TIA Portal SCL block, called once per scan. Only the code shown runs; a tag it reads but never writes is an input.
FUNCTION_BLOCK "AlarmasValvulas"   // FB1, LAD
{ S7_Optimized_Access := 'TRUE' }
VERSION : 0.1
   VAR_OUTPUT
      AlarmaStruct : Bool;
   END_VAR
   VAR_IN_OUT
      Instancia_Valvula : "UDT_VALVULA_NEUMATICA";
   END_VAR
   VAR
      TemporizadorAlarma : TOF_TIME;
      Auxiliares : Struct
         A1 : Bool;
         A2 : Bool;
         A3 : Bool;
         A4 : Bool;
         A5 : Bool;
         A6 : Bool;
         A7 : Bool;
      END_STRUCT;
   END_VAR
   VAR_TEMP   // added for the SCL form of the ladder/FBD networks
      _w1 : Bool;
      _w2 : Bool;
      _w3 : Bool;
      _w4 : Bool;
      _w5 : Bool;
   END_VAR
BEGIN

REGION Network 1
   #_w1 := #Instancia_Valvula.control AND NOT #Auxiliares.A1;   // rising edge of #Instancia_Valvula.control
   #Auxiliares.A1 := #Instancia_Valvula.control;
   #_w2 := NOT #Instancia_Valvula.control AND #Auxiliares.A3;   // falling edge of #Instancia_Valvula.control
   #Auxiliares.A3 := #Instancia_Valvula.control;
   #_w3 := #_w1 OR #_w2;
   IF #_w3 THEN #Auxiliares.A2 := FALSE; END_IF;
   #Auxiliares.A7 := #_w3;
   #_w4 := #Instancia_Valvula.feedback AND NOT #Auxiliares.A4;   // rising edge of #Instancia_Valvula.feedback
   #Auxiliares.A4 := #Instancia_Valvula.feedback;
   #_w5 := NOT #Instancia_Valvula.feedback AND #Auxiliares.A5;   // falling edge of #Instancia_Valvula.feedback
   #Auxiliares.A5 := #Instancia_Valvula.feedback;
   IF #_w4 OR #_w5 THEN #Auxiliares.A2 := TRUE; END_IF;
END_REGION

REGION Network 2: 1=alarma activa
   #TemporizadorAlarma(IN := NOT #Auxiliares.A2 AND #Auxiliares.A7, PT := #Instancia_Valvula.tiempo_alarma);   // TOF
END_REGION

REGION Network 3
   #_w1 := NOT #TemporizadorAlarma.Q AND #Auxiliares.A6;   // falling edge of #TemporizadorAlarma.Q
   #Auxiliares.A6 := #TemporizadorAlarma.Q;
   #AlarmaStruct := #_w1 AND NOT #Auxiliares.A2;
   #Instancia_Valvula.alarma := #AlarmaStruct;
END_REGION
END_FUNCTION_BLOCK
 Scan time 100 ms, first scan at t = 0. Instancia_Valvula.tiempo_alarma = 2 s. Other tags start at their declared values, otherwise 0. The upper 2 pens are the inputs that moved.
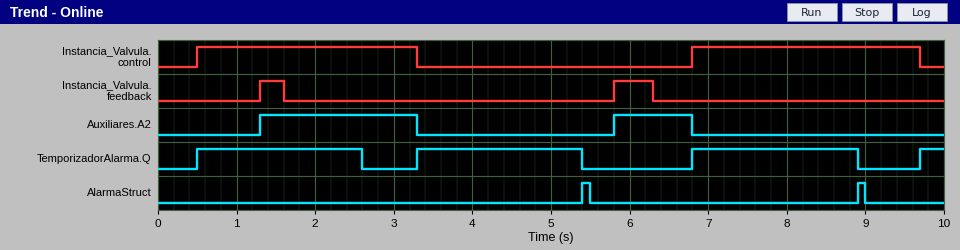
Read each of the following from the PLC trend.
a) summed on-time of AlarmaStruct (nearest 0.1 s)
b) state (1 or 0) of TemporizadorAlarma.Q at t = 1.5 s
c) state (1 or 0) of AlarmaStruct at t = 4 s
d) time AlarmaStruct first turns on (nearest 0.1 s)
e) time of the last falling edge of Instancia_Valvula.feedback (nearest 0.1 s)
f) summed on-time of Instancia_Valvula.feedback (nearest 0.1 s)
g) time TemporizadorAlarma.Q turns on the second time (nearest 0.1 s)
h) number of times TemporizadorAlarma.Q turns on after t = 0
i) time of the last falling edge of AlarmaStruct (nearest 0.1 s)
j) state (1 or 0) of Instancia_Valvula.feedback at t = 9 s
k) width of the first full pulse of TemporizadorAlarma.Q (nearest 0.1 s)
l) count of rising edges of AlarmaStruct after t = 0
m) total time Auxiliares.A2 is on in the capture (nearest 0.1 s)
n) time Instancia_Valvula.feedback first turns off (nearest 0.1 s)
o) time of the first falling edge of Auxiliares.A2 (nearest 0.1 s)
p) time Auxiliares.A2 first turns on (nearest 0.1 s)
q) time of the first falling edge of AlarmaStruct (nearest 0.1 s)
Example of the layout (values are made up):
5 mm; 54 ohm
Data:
0.2 s; 1; 0; 5.4 s; 6.3 s; 0.8 s; 3.3 s; 4; 9.0 s; 0; 2.1 s; 2; 3.0 s; 1.6 s; 3.3 s; 1.3 s; 5.5 s
